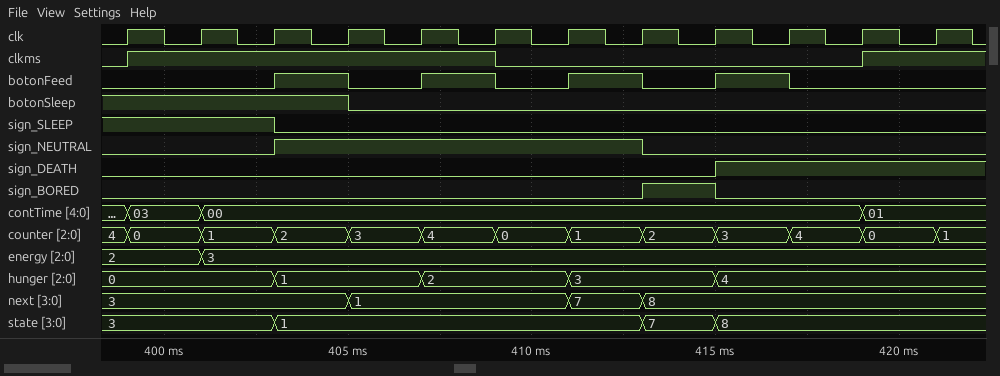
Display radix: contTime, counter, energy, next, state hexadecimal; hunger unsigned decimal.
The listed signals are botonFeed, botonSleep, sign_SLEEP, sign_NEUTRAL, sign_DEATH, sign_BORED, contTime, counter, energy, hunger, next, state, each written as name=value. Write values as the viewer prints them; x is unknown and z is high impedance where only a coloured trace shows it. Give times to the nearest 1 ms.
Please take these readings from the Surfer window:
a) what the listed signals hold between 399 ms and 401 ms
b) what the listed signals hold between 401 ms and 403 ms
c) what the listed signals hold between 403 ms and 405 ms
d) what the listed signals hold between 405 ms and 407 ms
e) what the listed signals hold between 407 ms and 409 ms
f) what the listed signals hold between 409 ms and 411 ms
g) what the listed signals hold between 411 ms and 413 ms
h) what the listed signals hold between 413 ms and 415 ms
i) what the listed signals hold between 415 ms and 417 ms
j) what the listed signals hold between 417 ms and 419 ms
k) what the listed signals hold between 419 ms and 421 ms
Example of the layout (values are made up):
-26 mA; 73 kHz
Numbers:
botonFeed=0, botonSleep=1, sign_SLEEP=1, sign_NEUTRAL=0, sign_DEATH=0, sign_BORED=0, contTime=03, counter=0, energy=2, hunger=0, next=3, state=3; botonFeed=0, botonSleep=1, sign_SLEEP=1, sign_NEUTRAL=0, sign_DEATH=0, sign_BORED=0, contTime=00, counter=1, energy=3, hunger=0, next=3, state=3; botonFeed=1, botonSleep=1, sign_SLEEP=0, sign_NEUTRAL=1, sign_DEATH=0, sign_BORED=0, contTime=00, counter=2, energy=3, hunger=1, next=3, state=1; botonFeed=0, botonSleep=0, sign_SLEEP=0, sign_NEUTRAL=1, sign_DEATH=0, sign_BORED=0, contTime=00, counter=3, energy=3, hunger=1, next=1, state=1; botonFeed=1, botonSleep=0, sign_SLEEP=0, sign_NEUTRAL=1, sign_DEATH=0, sign_BORED=0, contTime=00, counter=4, energy=3, hunger=2, next=1, state=1; botonFeed=0, botonSleep=0, sign_SLEEP=0, sign_NEUTRAL=1, sign_DEATH=0, sign_BORED=0, contTime=00, counter=0, energy=3, hunger=2, next=1, state=1; botonFeed=1, botonSleep=0, sign_SLEEP=0, sign_NEUTRAL=1, sign_DEATH=0, sign_BORED=0, contTime=00, counter=1, energy=3, hunger=3, next=7, state=1; botonFeed=0, botonSleep=0, sign_SLEEP=0, sign_NEUTRAL=0, sign_DEATH=0, sign_BORED=1, contTime=00, counter=2, energy=3, hunger=3, next=8, state=7; botonFeed=1, botonSleep=0, sign_SLEEP=0, sign_NEUTRAL=0, sign_DEATH=1, sign_BORED=0, contTime=00, counter=3, energy=3, hunger=4, next=8, state=8; botonFeed=0, botonSleep=0, sign_SLEEP=0, sign_NEUTRAL=0, sign_DEATH=1, sign_BORED=0, contTime=00, counter=4, energy=3, hunger=4, next=8, state=8; botonFeed=0, botonSleep=0, sign_SLEEP=0, sign_NEUTRAL=0, sign_DEATH=1, sign_BORED=0, contTime=01, counter=0, energy=3, hunger=4, next=8, state=8
